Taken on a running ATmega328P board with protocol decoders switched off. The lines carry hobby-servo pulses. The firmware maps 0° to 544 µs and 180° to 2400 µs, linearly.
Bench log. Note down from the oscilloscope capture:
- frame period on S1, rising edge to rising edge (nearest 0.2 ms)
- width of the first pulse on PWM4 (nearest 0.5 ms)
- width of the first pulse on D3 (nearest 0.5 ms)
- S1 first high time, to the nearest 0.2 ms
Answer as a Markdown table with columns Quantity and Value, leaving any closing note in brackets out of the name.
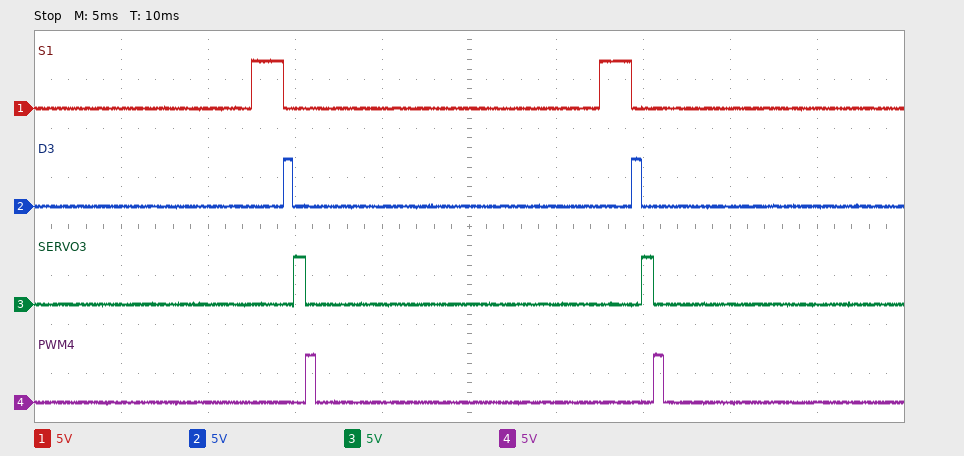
| Quantity | Value |
|---|---|
| frame period on S1, rising edge to rising edge | 20.0 ms |
| width of the first pulse on PWM4 | 0.5 ms |
| width of the first pulse on D3 | 0.5 ms |
| S1 first high time, to the nearest 0.2 ms | 1.8 ms |
